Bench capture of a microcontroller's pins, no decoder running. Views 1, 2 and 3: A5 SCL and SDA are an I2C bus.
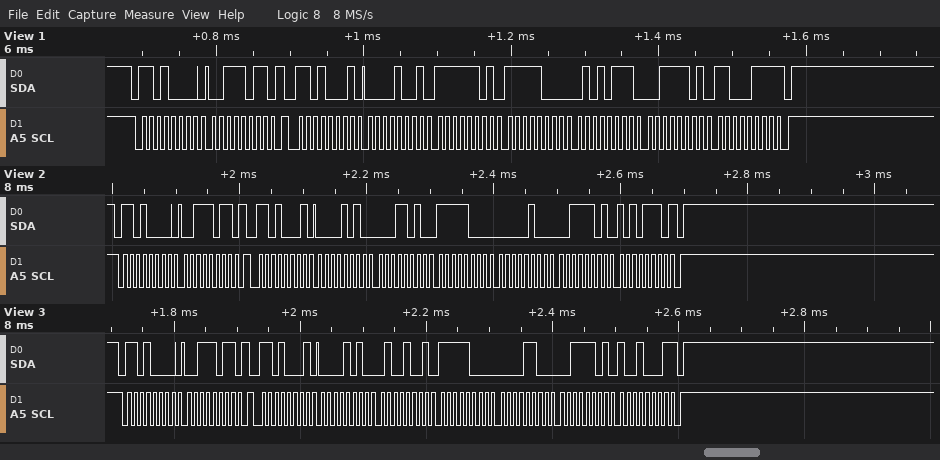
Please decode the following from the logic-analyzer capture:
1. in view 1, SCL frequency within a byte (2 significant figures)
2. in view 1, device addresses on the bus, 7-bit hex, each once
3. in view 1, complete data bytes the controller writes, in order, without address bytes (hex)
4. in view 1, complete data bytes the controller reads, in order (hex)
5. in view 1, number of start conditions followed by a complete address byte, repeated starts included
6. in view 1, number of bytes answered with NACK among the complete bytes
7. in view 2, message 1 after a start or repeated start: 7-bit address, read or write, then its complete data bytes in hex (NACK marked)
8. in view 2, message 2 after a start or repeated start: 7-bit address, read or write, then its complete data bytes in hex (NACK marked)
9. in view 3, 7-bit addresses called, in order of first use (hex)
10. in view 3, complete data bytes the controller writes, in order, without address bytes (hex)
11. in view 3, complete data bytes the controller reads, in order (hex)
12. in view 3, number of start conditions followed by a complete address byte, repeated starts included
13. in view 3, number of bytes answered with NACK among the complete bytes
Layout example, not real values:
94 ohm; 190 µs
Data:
100 kHz; 0x68; 3B; 09 FD F8 57 3D C7; 2; 1; 0x68 write: 3B; 0x68 read: 0A 1A F8 04 3D AE NACK; 0x68; 3B; 0A 49 F8 0C 3D 91; 2; 1
